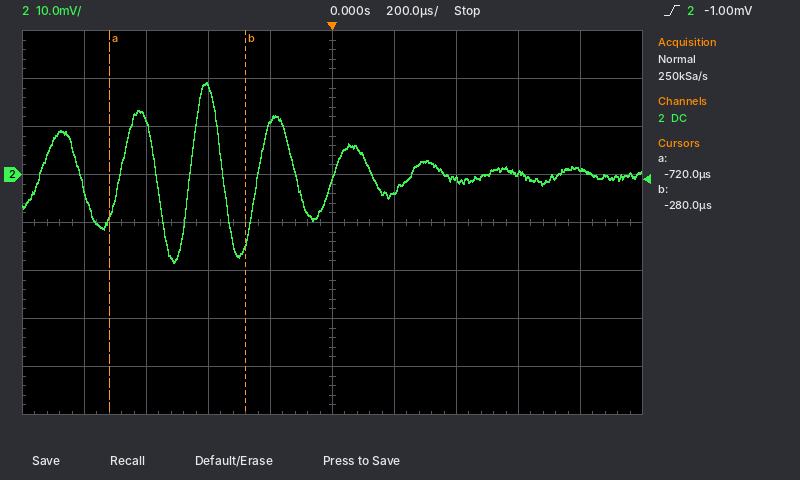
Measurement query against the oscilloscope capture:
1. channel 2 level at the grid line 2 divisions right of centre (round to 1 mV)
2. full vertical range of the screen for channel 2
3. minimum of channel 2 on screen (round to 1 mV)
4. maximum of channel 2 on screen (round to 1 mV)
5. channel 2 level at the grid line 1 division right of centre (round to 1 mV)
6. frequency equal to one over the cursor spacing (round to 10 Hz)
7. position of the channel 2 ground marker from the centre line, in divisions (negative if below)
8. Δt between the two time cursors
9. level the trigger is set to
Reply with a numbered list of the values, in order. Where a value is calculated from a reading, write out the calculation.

1. -1 mV
2. 80 mV
3. -18 mV
4. 19 mV
5. -4 mV
6. 1 / 440 µs ≈ 2.27 kHz
7. +1.0 div
8. -280 µs − (-720 µs) = 440 µs
9. -1.00 mV
